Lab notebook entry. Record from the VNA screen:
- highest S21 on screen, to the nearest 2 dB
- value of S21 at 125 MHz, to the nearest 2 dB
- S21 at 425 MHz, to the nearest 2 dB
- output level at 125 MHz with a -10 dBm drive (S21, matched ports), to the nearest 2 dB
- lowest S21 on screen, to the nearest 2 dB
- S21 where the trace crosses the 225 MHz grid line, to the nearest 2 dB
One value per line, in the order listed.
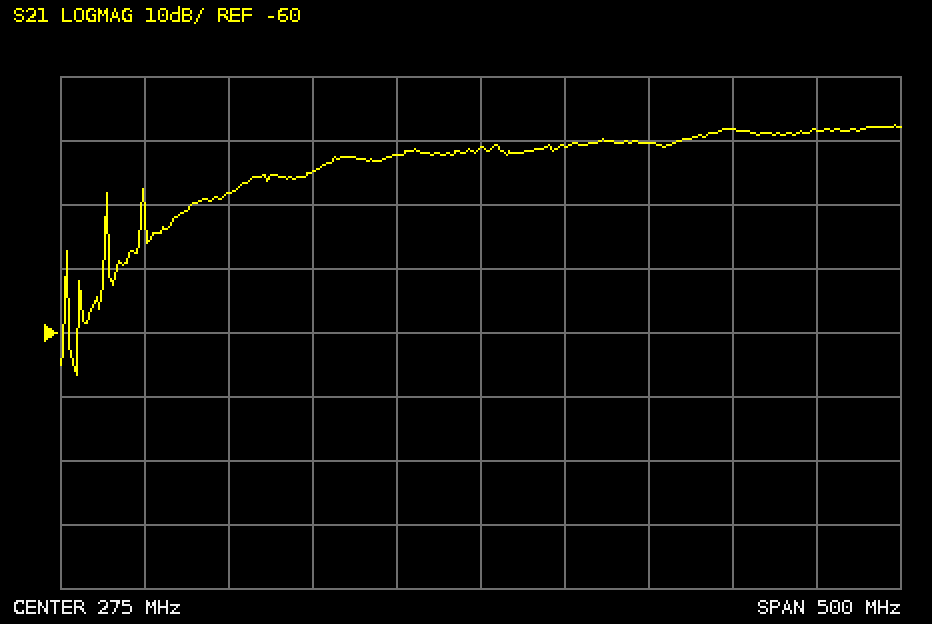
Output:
-28 dB
-38 dB
-28 dB
-48 dBm
-66 dB
-32 dB
